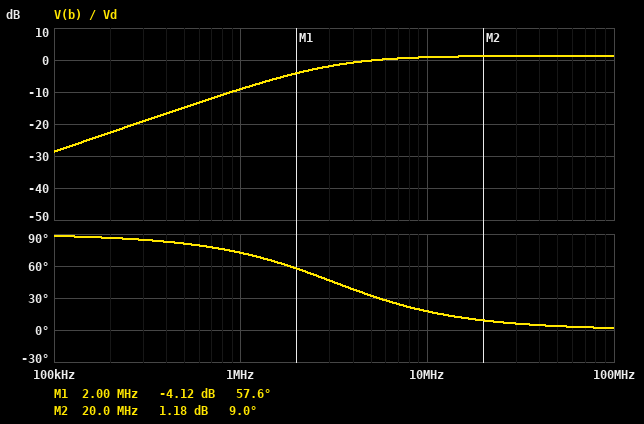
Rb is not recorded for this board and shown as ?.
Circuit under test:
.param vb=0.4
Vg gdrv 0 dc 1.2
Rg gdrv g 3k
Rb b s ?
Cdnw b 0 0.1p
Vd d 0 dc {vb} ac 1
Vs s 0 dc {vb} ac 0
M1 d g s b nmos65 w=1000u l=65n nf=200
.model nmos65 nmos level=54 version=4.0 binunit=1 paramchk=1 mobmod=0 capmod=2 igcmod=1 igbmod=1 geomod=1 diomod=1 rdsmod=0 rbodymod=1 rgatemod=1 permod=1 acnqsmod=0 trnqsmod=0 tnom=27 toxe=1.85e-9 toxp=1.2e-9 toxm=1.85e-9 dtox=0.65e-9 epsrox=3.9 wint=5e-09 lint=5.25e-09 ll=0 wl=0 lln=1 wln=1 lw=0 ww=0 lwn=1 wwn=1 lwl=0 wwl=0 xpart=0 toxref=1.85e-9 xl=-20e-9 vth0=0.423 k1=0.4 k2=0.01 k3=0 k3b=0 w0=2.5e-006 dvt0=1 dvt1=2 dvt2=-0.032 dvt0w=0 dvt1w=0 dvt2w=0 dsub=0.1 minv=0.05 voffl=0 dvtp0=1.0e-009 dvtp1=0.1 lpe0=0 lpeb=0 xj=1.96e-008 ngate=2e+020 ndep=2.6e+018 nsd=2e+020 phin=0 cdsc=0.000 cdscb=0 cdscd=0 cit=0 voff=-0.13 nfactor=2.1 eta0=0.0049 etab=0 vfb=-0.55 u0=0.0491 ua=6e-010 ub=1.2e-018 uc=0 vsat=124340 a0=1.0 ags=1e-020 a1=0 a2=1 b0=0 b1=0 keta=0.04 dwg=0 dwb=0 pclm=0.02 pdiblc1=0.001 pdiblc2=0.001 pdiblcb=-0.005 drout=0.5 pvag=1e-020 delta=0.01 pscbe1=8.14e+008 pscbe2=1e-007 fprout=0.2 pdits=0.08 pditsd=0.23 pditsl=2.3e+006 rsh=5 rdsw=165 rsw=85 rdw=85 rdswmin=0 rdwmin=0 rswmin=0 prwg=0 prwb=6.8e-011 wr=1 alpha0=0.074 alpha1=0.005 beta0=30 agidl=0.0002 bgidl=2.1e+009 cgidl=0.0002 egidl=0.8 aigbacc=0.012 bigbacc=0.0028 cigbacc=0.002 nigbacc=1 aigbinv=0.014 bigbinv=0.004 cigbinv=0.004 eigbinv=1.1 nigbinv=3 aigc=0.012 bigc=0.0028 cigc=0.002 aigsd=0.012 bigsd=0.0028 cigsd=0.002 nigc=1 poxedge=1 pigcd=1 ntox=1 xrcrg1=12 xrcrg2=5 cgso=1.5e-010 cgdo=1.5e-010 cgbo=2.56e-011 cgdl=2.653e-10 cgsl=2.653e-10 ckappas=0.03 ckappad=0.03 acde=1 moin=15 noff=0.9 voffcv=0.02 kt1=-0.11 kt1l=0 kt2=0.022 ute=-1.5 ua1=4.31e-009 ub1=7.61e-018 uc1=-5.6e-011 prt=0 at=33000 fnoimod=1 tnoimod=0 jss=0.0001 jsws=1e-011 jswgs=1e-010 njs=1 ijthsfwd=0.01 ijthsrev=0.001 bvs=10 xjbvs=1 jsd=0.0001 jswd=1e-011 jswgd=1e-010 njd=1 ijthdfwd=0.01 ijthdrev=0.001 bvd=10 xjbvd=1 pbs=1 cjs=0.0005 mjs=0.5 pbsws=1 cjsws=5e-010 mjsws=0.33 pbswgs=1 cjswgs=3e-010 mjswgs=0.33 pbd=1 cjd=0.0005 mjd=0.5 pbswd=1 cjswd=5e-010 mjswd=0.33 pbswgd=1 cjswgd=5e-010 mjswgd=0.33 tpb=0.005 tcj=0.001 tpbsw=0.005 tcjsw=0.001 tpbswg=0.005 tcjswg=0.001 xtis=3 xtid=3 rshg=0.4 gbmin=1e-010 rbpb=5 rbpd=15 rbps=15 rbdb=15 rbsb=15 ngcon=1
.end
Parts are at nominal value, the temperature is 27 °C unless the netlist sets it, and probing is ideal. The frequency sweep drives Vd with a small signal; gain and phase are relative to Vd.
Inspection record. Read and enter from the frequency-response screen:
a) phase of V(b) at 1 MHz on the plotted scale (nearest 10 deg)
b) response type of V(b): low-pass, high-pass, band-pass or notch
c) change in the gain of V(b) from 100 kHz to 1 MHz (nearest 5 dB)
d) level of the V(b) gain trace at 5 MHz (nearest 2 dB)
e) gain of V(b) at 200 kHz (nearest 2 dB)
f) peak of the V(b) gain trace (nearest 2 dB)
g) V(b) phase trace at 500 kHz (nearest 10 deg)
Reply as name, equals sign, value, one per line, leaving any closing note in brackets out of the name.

phase of V(b) at 1 MHz on the plotted scale = 70 deg
response type of V(b): low-pass, high-pass, band-pass or notch = high-pass
change in the gain of V(b) from 100 kHz to 1 MHz = 20 dB
level of the V(b) gain trace at 5 MHz = 0 dB
gain of V(b) at 200 kHz = -22 dB
peak of the V(b) gain trace = 2 dB
V(b) phase trace at 500 kHz = 80 deg
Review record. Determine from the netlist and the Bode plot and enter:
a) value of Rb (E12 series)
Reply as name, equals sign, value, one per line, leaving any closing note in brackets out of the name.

value of Rb = 47 kΩ
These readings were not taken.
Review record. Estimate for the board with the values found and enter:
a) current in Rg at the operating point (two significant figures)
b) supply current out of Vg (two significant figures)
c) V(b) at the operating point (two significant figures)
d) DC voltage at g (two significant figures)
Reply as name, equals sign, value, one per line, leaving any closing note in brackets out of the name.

current in Rg at the operating point = 2.8 µA
supply current out of Vg = 2.8 µA
V(b) at the operating point = 400 mV
DC voltage at g = 1.2 V
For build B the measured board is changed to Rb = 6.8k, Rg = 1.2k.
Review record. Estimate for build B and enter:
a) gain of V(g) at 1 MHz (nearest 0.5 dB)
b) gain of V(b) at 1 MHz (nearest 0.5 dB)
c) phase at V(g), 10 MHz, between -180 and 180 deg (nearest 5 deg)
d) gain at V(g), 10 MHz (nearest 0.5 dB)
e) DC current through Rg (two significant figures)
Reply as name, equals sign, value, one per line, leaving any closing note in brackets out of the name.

gain of V(g) at 1 MHz = -42.0 dB
gain of V(b) at 1 MHz = -25.5 dB
phase at V(g), 10 MHz, between -180 and 180 deg = 80 deg
gain at V(g), 10 MHz = -24.0 dB
DC current through Rg = 2.9 µA
